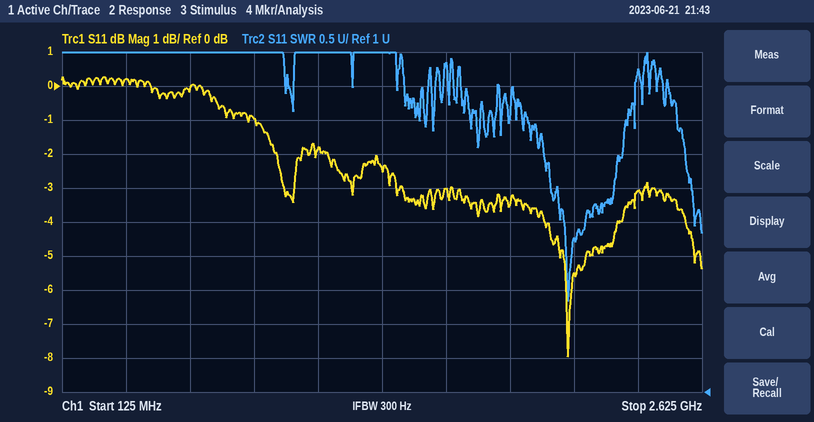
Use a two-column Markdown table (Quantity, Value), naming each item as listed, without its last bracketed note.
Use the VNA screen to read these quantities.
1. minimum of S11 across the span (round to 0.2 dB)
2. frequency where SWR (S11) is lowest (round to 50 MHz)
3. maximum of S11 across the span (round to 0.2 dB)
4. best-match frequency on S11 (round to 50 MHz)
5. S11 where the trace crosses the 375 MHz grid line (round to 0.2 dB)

| Quantity | Value |
|---|---|
| minimum of S11 across the span | -8.0 dB |
| frequency where SWR (S11) is lowest | 2.10 GHz |
| maximum of S11 across the span | 0.2 dB |
| best-match frequency on S11 | 2.10 GHz |
| S11 where the trace crosses the 375 MHz grid line | 0.2 dB |
